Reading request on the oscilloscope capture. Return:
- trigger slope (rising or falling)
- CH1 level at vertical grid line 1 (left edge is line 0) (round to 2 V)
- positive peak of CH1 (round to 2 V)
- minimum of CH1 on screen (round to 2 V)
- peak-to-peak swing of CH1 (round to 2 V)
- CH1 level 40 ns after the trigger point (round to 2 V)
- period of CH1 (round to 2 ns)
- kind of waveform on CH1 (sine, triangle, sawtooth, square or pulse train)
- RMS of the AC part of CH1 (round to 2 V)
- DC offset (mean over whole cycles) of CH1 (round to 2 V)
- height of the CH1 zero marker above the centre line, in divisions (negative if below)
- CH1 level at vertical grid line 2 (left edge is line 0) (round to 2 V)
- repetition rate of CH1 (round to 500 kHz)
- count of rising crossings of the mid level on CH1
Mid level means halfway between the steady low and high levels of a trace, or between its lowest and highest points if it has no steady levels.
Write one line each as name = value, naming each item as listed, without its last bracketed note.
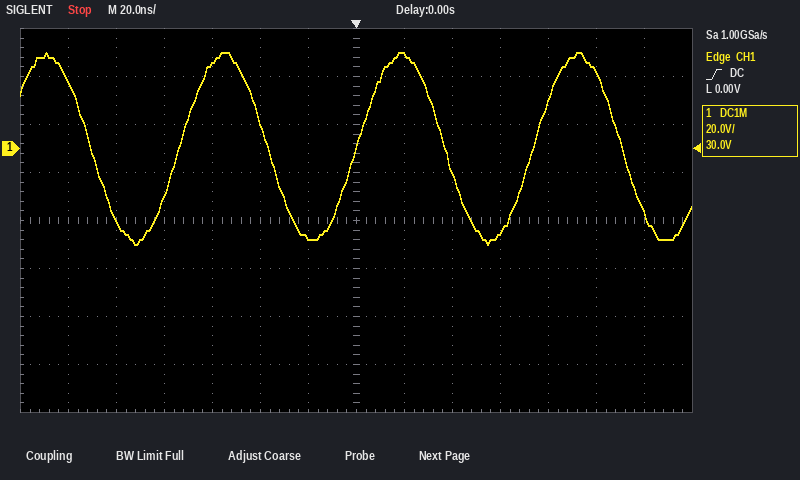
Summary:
trigger slope = rising
CH1 level at vertical grid line 1 (left edge is line 0) = 28 V
positive peak of CH1 = 40 V
minimum of CH1 on screen = -40 V
peak-to-peak swing of CH1 = 80 V
CH1 level 40 ns after the trigger point = -10 V
period of CH1 = 74 ns
kind of waveform on CH1 = sine
RMS of the AC part of CH1 = 28 V
DC offset (mean over whole cycles) of CH1 = 0 V
height of the CH1 zero marker above the centre line, in divisions = +1.5 div
CH1 level at vertical grid line 2 (left edge is line 0) = -30 V
repetition rate of CH1 = 13.5 MHz
count of rising crossings of the mid level on CH1 = 3
